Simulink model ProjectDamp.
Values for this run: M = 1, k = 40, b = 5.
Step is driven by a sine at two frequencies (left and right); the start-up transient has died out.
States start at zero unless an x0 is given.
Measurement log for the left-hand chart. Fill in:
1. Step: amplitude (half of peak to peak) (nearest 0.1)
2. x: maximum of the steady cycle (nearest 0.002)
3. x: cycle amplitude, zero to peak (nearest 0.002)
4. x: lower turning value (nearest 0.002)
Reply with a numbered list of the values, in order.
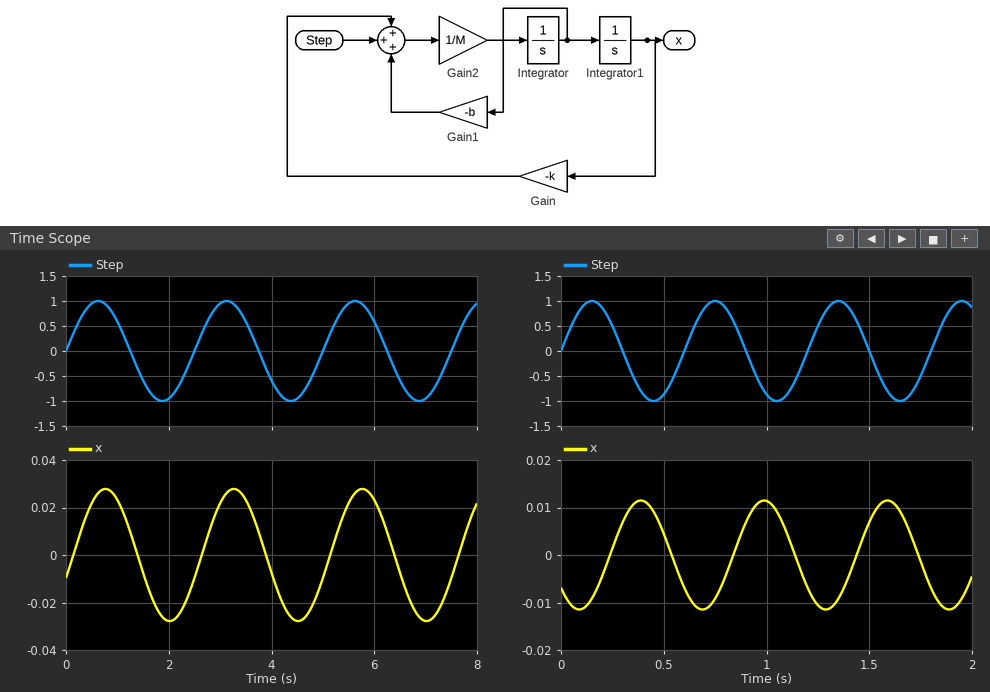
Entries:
1. 1.0
2. 0.028
3. 0.028
4. -0.028
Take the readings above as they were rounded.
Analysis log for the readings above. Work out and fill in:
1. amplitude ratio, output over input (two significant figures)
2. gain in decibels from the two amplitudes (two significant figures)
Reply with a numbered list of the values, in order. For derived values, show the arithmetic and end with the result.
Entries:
1. 0.028 / 1 = 0.028
2. 20 log10(0.028 / 1) = -31 dB
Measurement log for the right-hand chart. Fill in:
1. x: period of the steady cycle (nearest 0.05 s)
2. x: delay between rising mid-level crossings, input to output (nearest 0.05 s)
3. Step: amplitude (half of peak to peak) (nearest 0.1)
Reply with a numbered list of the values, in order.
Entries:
1. 0.60 s
2. 0.25 s
3. 1.0
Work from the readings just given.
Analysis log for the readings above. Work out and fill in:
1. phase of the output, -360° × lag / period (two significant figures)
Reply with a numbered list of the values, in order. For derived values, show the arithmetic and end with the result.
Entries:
1. -360 × 0.25 / 0.6 = -150°
